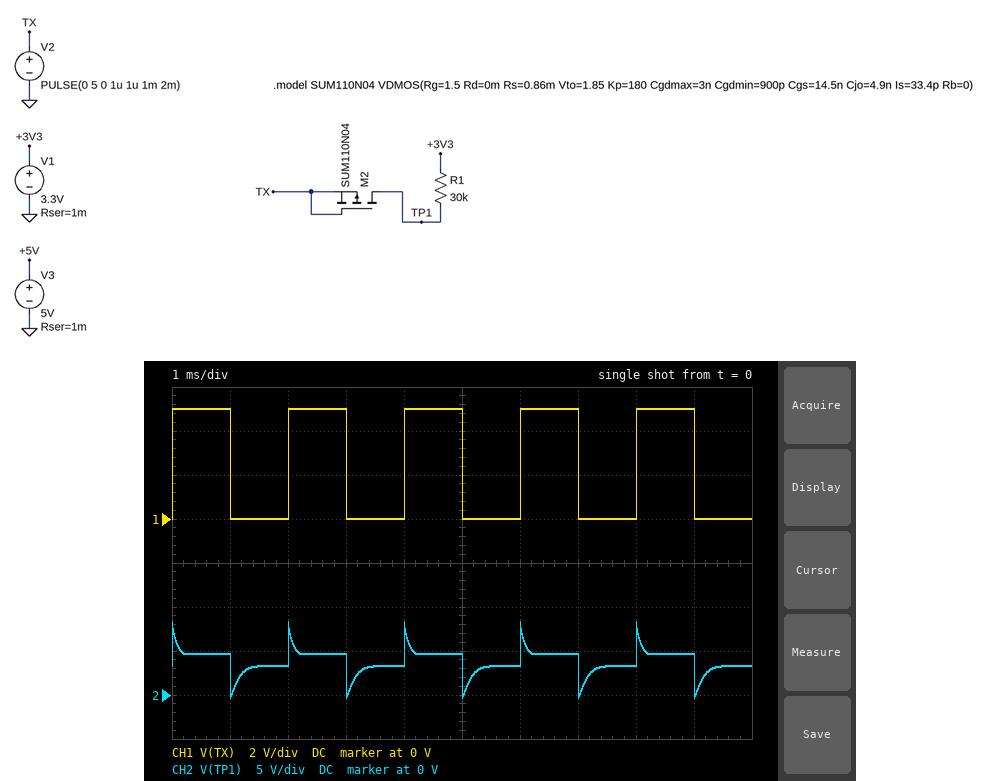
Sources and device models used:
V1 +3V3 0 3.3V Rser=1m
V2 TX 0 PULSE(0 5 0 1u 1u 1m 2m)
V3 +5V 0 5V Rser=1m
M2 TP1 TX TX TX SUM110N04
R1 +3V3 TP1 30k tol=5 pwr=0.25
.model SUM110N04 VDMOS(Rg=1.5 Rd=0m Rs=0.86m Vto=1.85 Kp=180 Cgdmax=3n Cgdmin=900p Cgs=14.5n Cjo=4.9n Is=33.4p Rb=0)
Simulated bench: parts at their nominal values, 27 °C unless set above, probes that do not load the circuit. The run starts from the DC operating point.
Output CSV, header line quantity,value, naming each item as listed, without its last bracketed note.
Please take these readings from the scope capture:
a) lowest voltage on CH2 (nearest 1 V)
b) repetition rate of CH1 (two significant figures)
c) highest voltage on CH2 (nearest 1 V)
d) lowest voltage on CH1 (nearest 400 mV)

quantity,value
lowest voltage on CH2,0 V
repetition rate of CH1,500 Hz
highest voltage on CH2,8 V
lowest voltage on CH1,0 V
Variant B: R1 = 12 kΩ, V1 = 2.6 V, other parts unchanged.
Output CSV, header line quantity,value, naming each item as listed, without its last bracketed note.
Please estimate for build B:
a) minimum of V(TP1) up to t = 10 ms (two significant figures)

quantity,value
minimum of V(TP1) up to t = 10 ms,-380 mV
